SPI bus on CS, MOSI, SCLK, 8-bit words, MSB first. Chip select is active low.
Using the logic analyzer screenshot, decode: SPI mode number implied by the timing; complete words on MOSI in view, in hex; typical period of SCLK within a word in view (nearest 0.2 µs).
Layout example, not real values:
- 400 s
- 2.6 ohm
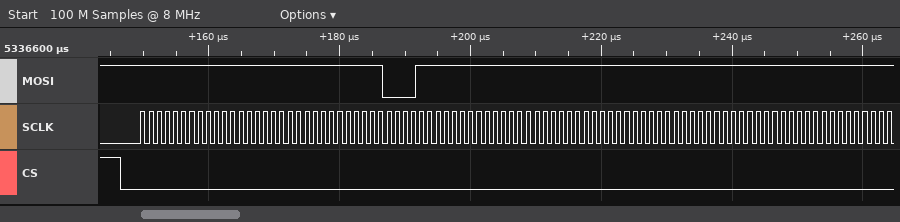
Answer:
- 0
- FF, FF, FF, FC, 3F, FF, FF, FF, FF, FF, FF
- 1.2 µs
